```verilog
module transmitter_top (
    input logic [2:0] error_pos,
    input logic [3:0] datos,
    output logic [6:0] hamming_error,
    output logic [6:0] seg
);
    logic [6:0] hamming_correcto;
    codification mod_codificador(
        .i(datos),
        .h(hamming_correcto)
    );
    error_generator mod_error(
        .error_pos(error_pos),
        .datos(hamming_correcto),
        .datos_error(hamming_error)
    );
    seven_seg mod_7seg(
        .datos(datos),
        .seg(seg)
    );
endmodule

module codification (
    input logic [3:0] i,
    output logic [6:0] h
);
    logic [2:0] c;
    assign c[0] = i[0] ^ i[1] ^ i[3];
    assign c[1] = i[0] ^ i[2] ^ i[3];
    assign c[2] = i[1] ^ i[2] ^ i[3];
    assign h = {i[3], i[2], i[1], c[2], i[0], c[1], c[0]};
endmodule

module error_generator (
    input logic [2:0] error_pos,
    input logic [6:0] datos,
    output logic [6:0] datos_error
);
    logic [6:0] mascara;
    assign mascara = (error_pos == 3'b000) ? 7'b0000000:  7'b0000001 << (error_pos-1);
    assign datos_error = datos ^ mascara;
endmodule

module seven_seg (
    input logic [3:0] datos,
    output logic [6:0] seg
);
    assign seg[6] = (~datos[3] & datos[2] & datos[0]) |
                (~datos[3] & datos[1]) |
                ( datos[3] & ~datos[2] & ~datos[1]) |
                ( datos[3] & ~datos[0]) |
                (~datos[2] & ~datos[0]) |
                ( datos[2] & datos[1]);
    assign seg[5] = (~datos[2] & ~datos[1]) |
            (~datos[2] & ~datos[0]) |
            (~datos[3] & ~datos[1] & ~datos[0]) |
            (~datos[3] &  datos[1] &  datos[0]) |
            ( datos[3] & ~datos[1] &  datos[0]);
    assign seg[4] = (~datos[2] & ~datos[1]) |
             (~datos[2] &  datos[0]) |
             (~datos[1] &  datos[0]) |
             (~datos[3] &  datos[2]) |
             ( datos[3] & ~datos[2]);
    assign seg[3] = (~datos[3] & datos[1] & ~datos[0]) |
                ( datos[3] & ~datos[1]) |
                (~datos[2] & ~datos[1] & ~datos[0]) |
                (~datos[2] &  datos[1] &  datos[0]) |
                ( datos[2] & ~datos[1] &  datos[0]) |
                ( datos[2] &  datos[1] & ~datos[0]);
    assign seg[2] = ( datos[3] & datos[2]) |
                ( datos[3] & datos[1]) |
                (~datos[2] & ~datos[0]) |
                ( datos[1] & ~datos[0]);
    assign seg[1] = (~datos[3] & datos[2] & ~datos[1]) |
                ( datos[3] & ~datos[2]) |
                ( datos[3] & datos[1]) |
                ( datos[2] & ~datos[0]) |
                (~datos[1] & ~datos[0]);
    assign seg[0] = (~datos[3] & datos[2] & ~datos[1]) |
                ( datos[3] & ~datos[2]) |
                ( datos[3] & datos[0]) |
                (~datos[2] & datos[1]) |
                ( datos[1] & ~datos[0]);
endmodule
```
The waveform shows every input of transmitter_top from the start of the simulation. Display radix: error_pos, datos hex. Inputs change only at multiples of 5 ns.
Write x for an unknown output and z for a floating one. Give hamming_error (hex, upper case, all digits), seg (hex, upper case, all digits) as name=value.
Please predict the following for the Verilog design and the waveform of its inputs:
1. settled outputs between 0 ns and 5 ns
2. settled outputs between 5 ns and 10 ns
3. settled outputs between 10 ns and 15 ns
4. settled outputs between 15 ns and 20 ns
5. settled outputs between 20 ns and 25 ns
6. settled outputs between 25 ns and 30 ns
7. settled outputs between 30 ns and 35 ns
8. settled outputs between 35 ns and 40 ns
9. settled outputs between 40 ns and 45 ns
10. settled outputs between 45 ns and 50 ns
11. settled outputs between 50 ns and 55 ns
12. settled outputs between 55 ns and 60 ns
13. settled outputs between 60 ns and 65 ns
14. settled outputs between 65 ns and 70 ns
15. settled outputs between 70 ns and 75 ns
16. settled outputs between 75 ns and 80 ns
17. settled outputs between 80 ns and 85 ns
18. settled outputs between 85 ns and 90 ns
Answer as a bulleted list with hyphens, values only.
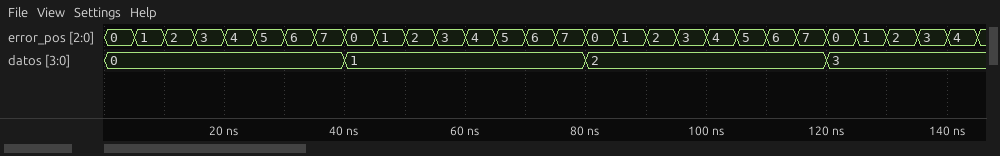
- hamming_error=00, seg=7E
- hamming_error=01, seg=7E
- hamming_error=02, seg=7E
- hamming_error=04, seg=7E
- hamming_error=08, seg=7E
- hamming_error=10, seg=7E
- hamming_error=20, seg=7E
- hamming_error=40, seg=7E
- hamming_error=07, seg=30
- hamming_error=06, seg=30
- hamming_error=05, seg=30
- hamming_error=03, seg=30
- hamming_error=0F, seg=30
- hamming_error=17, seg=30
- hamming_error=27, seg=30
- hamming_error=47, seg=30
- hamming_error=19, seg=6D
- hamming_error=18, seg=6D
